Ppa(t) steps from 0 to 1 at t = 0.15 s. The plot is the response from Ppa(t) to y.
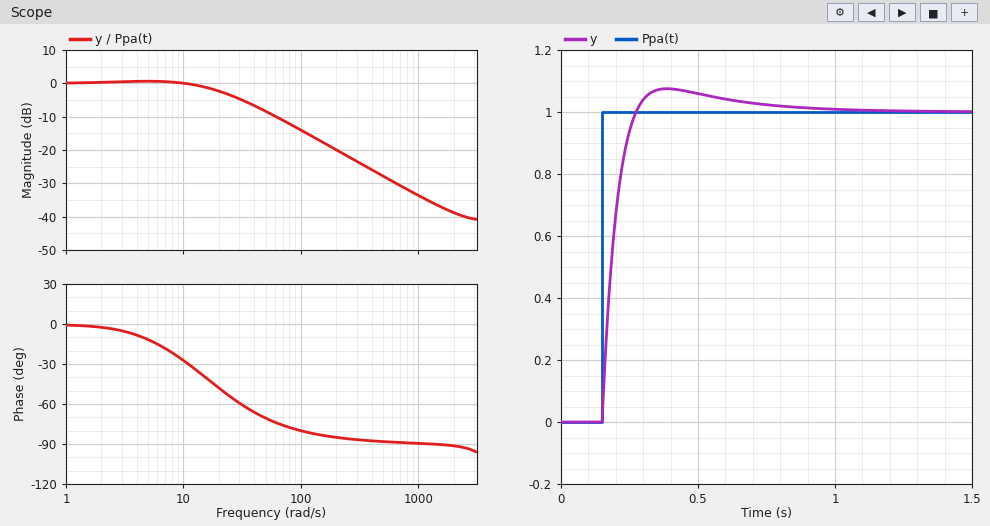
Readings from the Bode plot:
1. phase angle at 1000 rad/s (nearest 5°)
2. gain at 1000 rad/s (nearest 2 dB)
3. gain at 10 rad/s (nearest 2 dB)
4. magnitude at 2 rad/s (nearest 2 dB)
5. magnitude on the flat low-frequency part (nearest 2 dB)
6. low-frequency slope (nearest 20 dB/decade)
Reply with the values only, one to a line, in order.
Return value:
-90°
-34 dB
0 dB
0 dB
0 dB
0 dB/decade
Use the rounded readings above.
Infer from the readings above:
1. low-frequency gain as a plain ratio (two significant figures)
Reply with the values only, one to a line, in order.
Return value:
1.0
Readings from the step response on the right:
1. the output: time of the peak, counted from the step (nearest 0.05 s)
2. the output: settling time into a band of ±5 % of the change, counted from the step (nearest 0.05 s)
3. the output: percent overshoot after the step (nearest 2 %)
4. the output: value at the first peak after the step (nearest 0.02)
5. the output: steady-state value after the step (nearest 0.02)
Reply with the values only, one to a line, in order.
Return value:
0.25 s
0.40 s
8 %
1.08
1.00
